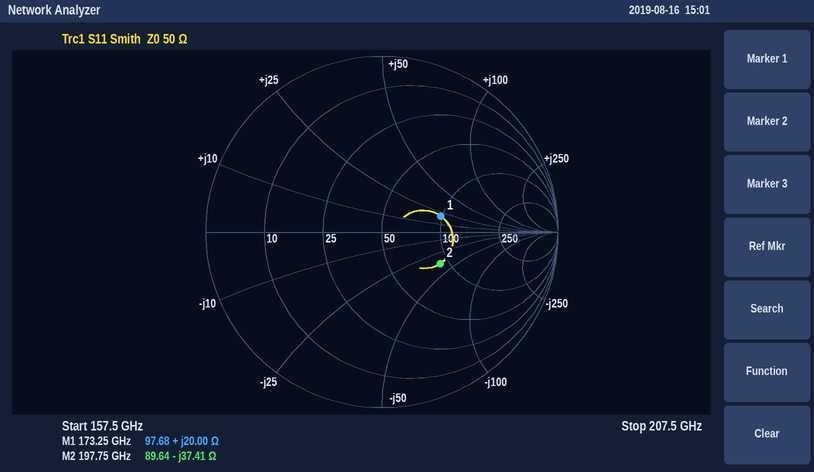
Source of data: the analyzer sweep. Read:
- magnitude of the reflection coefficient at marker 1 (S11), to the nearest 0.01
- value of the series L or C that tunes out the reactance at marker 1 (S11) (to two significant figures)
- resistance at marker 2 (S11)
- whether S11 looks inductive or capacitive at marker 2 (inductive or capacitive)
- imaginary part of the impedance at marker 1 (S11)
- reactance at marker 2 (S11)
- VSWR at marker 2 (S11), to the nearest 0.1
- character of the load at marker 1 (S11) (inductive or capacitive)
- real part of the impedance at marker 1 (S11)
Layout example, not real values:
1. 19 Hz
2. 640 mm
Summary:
1. 0.35
2. 46 fF
3. 89.64 Ω
4. capacitive
5. +20.00 Ω
6. -37.41 Ω
7. 2.2
8. inductive
9. 97.68 Ω
